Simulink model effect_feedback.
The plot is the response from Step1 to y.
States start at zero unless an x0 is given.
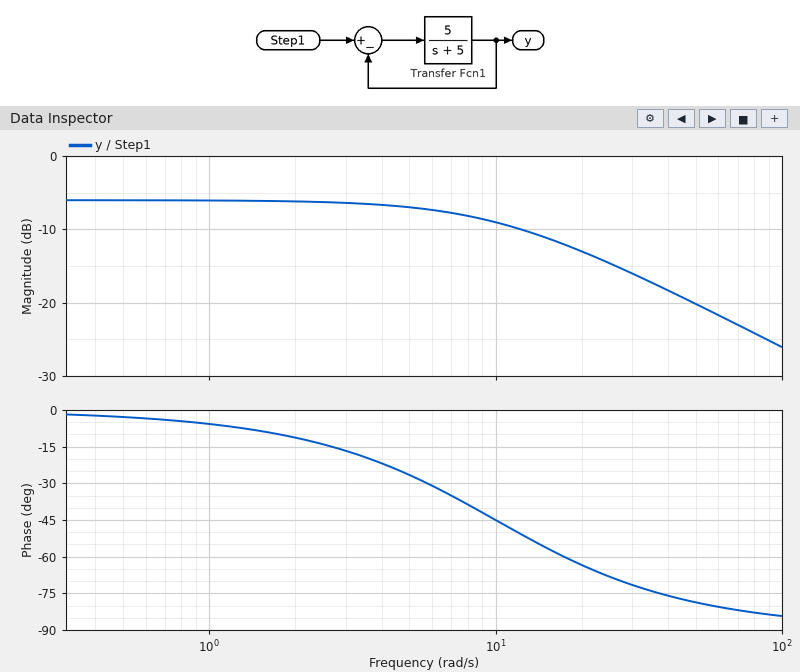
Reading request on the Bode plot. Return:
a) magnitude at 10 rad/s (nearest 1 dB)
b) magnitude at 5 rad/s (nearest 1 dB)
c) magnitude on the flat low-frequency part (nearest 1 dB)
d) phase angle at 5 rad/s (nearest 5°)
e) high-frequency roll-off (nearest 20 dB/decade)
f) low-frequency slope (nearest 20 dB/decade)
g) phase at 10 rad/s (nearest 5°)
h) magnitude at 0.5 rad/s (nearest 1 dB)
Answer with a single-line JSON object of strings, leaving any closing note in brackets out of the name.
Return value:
{"magnitude at 10 rad/s": "-9 dB", "magnitude at 5 rad/s": "-7 dB", "magnitude on the flat low-frequency part": "-6 dB", "phase angle at 5 rad/s": "-25°", "high-frequency roll-off": "-20 dB/decade", "low-frequency slope": "0 dB/decade", "phase at 10 rad/s": "-45°", "magnitude at 0.5 rad/s": "-6 dB"}
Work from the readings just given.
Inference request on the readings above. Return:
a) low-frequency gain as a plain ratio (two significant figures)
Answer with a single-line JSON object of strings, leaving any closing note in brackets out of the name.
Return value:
{"low-frequency gain as a plain ratio": "0.50"}
